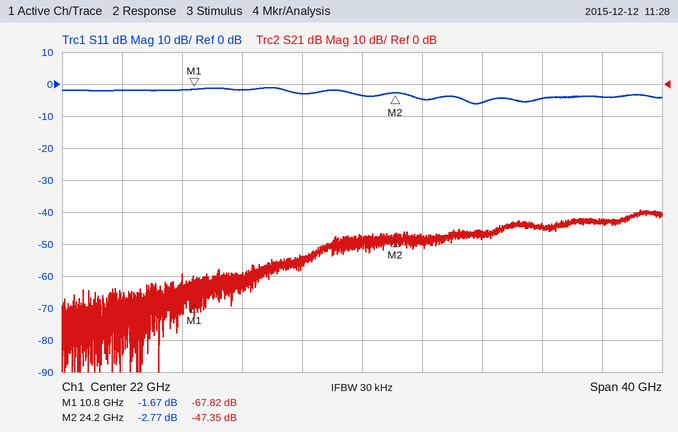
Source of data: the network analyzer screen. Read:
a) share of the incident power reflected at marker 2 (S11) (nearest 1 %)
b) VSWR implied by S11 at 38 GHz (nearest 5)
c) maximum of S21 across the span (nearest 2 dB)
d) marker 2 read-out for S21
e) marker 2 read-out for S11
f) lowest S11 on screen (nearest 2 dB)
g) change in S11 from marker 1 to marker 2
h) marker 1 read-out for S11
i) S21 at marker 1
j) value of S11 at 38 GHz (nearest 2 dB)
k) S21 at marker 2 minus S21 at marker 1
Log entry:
53 %
5
-40 dB
-47.35 dB
-2.77 dB
-6 dB
-1.10 dB
-1.67 dB
-67.82 dB
-4 dB
20.47 dB
